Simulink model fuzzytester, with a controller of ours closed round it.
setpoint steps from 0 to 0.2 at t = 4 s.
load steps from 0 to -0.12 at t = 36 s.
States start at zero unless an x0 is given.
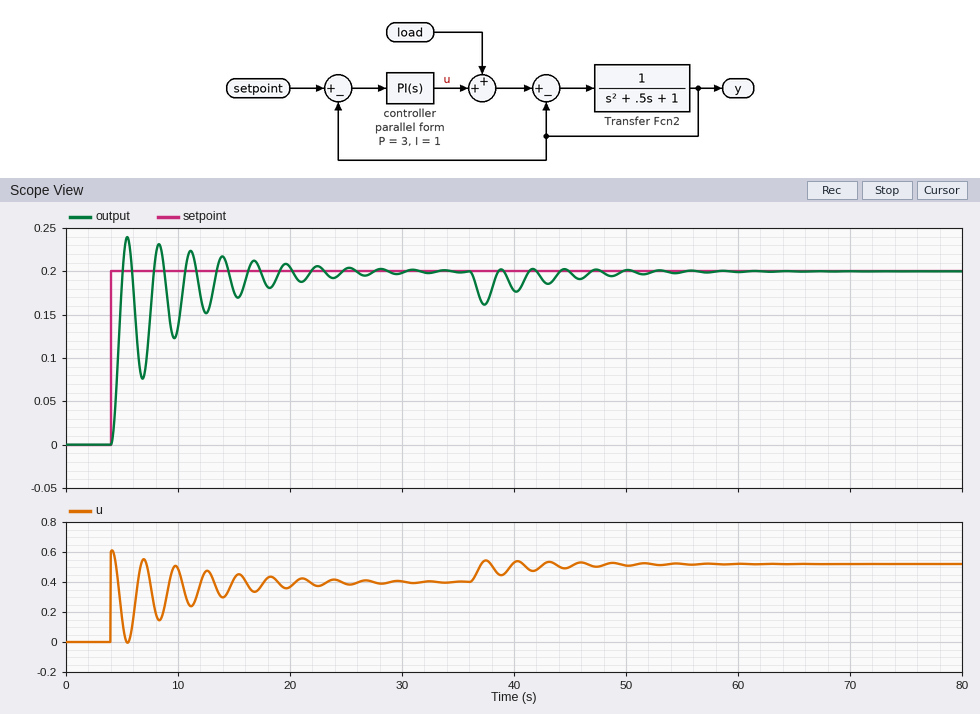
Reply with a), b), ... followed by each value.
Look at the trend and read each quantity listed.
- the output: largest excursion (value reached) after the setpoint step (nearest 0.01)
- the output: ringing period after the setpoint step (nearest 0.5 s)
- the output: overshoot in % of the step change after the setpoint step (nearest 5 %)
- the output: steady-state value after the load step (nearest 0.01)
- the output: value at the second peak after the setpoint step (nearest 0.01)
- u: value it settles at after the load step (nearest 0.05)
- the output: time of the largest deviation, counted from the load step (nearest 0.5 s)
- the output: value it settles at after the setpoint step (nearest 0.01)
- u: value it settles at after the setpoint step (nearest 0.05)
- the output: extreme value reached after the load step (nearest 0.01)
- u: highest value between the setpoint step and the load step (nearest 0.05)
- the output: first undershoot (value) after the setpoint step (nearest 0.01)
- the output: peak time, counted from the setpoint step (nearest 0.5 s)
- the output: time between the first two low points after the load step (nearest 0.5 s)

a) 0.24
b) 3.0 s
c) 20 %
d) 0.20
e) 0.23
f) 0.50
g) 1.5 s
h) 0.20
i) 0.40
j) 0.16
k) 0.60
l) 0.08
m) 1.5 s
n) 3.0 s
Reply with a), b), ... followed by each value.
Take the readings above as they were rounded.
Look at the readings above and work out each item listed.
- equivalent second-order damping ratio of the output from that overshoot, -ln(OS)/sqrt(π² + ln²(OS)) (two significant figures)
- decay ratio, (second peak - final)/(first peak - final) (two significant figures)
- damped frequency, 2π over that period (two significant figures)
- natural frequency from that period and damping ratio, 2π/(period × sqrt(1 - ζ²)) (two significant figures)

a) 0.46
b) 0.75
c) 2.1 rad/s
d) 2.4 rad/s
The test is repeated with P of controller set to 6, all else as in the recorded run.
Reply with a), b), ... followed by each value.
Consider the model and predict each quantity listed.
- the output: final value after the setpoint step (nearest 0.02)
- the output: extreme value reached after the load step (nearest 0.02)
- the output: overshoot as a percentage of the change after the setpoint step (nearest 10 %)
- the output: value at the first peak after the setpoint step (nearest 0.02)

a) 0.20
b) 0.18
c) 40 %
d) 0.28
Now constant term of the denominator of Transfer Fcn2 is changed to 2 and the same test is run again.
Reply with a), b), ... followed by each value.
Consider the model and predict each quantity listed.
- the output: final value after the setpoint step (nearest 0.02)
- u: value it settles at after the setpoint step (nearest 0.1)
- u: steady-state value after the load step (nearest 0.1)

a) 0.20
b) 0.6
c) 0.7
